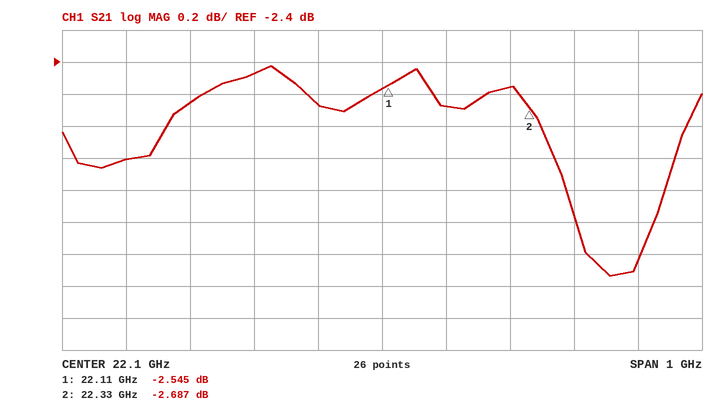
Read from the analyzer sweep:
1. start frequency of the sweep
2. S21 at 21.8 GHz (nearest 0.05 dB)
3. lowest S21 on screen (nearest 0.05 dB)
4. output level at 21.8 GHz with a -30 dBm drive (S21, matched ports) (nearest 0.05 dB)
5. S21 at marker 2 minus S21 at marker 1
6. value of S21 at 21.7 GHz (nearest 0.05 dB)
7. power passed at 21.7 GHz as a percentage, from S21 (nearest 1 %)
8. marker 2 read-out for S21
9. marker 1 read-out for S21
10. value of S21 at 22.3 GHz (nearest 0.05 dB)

21.6 GHz
-2.65 dB
-3.75 dB
-32.65 dBm
-0.142 dB
-3.00 dB
50 %
-2.687 dB
-2.545 dB
-2.55 dB
